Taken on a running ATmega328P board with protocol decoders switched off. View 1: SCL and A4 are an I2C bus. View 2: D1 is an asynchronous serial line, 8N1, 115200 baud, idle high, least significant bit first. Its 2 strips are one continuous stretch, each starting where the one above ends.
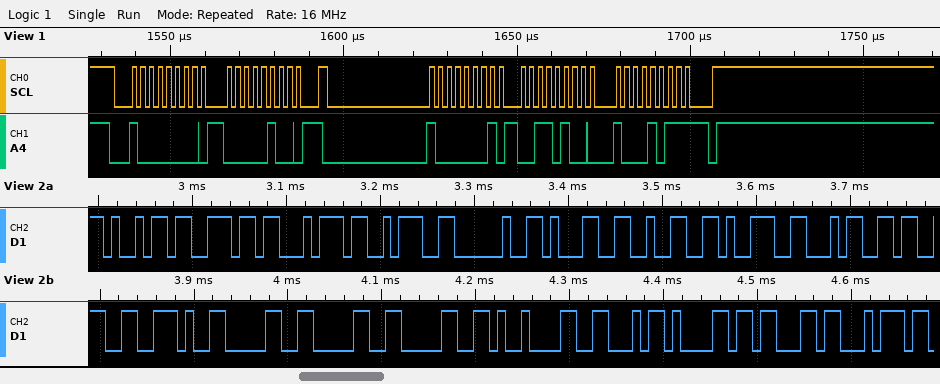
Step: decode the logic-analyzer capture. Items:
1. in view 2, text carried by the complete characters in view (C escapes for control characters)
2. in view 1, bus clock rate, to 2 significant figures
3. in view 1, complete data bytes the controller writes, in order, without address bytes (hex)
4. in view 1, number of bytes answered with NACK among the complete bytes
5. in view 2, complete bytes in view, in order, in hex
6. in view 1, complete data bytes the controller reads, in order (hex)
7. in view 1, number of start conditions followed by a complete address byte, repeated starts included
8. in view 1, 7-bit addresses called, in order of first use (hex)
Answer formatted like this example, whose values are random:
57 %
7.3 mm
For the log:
"int: 12943.000\tFact"
400 kHz
04
1
69 6E 74 3A 20 31 32 39 34 33 2E 30 30 30 09 46 61 63 74
34 8B
2
0x40
